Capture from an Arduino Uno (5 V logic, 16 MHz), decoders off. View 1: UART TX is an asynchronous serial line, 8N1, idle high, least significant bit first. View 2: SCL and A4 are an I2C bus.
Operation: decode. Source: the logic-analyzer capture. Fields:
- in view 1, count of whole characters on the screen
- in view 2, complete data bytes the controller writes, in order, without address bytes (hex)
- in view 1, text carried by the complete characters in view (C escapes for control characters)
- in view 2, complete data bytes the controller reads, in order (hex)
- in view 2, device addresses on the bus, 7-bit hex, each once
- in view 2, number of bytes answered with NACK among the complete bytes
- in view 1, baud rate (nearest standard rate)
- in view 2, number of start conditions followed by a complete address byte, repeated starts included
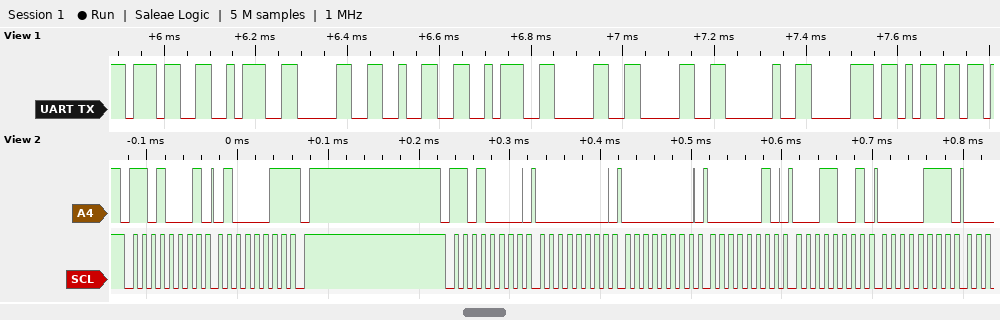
10
00 00 02 19 07
"7:02:00 pm"
43
0x68
1
57600 baud
2
